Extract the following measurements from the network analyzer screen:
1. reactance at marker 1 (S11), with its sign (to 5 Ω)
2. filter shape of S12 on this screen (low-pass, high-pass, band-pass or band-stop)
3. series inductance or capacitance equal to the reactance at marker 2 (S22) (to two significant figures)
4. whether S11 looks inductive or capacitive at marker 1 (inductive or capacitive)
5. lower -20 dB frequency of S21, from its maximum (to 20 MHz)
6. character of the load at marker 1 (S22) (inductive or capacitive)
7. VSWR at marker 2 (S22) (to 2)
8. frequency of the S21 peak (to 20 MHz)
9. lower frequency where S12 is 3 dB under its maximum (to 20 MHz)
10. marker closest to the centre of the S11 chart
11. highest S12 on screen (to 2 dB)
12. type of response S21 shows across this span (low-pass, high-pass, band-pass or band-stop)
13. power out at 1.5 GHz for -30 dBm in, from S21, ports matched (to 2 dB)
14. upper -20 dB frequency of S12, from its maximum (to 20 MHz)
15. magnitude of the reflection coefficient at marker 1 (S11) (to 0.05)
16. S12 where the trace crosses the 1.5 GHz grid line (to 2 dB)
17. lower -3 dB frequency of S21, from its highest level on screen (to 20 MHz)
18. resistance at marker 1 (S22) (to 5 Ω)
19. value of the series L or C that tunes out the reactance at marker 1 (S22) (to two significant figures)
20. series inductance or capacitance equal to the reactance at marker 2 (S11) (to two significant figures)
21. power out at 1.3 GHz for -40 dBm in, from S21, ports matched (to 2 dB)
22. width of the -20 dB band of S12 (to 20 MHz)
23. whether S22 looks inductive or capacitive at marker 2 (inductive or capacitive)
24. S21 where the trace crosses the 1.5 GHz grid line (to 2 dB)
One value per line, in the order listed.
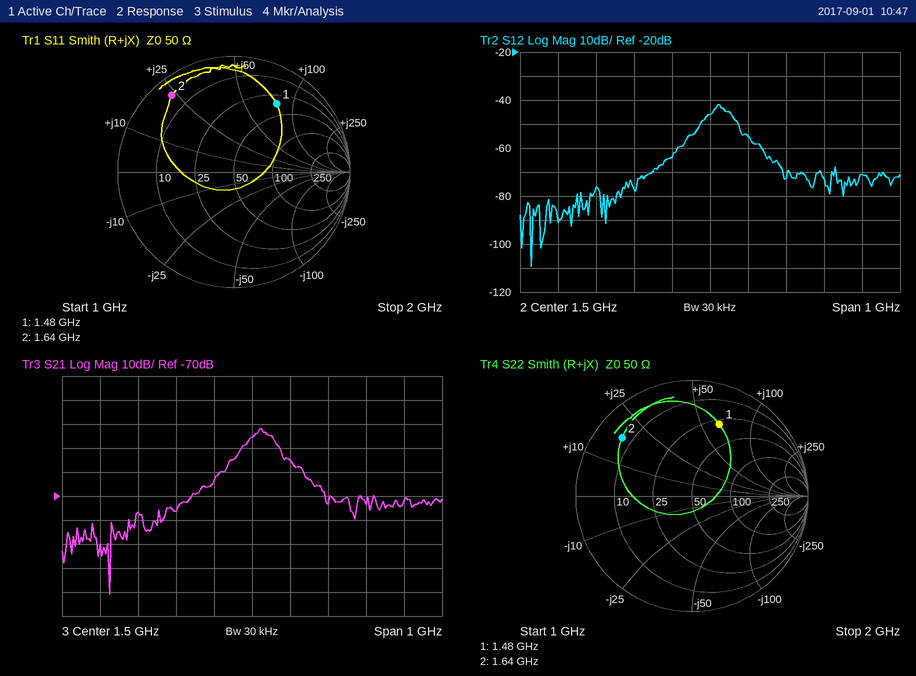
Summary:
+80 Ω
band-pass
1.7 nH
inductive
1.40 GHz
inductive
8
1.52 GHz
1.50 GHz
marker 1
-42 dB
band-pass
-76 dBm
1.64 GHz
0.70
-46 dB
1.50 GHz
30 Ω
1.7 pF
2.3 nH
-116 dBm
240 MHz
inductive
-46 dB
